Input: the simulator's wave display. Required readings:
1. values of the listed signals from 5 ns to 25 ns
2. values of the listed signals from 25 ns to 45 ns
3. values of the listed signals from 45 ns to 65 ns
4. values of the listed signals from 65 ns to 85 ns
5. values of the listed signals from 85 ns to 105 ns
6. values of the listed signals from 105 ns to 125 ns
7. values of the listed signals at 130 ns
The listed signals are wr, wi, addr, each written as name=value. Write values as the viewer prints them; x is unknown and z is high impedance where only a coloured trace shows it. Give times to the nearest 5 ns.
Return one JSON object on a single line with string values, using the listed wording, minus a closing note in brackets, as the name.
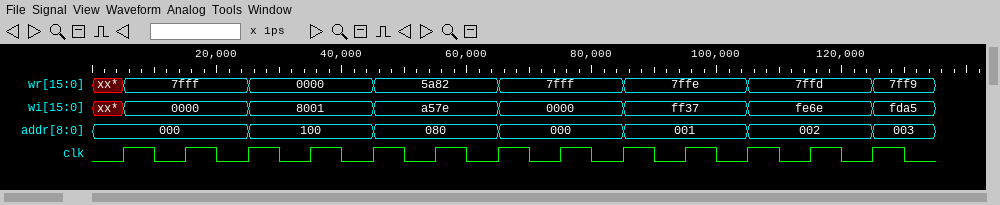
{"values of the listed signals from 5 ns to 25 ns": "wr=7fff, wi=0000, addr=000", "values of the listed signals from 25 ns to 45 ns": "wr=0000, wi=8001, addr=100", "values of the listed signals from 45 ns to 65 ns": "wr=5a82, wi=a57e, addr=080", "values of the listed signals from 65 ns to 85 ns": "wr=7fff, wi=0000, addr=000", "values of the listed signals from 85 ns to 105 ns": "wr=7ffe, wi=ff37, addr=001", "values of the listed signals from 105 ns to 125 ns": "wr=7ffd, wi=fe6e, addr=002", "values of the listed signals at 130 ns": "wr=7ff9, wi=fda5, addr=003"}
